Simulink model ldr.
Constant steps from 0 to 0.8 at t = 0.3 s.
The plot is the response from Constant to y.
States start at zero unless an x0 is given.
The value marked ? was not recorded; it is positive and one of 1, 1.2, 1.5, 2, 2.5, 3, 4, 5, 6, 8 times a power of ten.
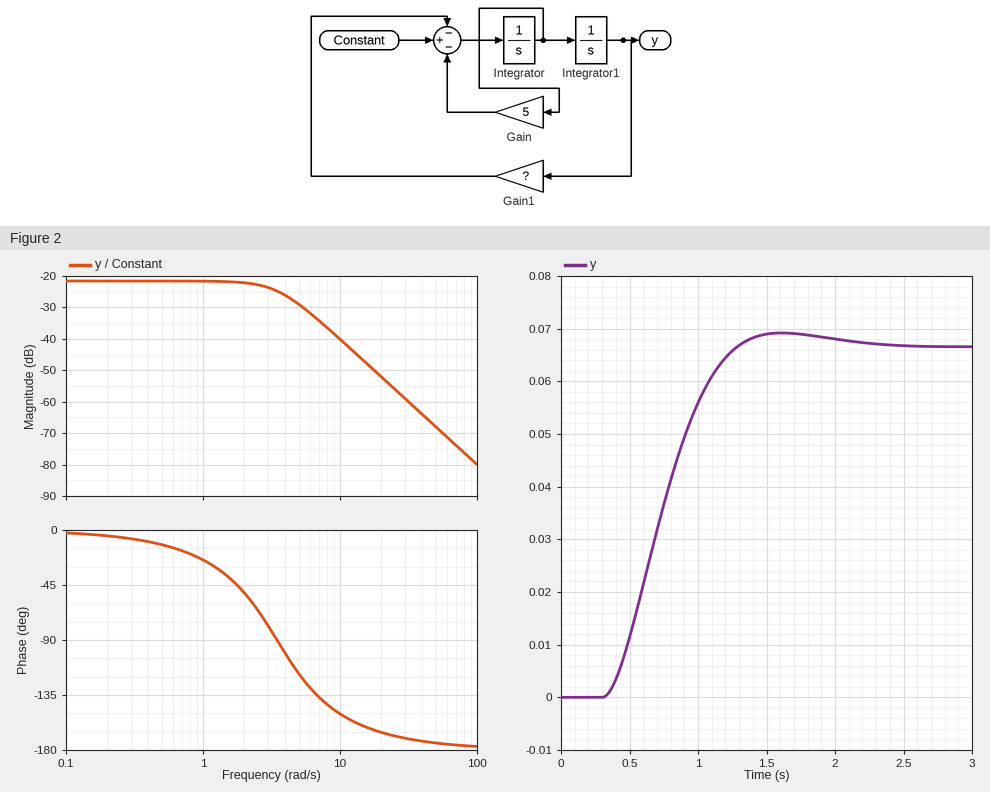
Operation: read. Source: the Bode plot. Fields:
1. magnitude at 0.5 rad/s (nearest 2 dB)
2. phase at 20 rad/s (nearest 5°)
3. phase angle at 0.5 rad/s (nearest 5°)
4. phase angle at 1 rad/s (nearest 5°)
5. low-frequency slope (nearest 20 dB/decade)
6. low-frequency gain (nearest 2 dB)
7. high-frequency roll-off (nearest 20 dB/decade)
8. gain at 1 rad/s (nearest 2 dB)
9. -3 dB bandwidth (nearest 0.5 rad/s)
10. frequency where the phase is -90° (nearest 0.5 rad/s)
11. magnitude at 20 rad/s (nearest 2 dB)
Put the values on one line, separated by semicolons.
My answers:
-22 dB; -165°; -10°; -25°; 0 dB/decade; -22 dB; -40 dB/decade; -22 dB; 3.5 rad/s; 3.5 rad/s; -52 dB
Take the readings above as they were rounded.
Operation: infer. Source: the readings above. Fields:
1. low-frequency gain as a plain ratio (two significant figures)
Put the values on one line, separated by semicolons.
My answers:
0.079
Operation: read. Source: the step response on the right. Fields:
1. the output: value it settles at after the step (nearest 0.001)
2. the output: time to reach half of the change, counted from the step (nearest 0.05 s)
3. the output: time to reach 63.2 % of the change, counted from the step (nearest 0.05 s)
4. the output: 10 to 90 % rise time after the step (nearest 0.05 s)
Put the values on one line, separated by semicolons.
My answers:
0.067; 0.40 s; 0.50 s; 0.65 s
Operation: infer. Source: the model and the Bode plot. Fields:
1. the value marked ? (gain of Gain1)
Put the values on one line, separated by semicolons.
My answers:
12
